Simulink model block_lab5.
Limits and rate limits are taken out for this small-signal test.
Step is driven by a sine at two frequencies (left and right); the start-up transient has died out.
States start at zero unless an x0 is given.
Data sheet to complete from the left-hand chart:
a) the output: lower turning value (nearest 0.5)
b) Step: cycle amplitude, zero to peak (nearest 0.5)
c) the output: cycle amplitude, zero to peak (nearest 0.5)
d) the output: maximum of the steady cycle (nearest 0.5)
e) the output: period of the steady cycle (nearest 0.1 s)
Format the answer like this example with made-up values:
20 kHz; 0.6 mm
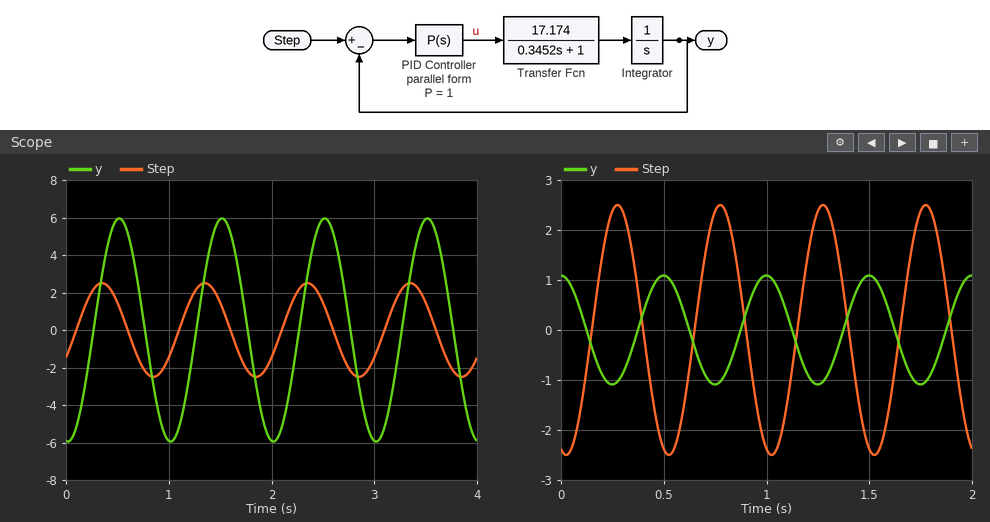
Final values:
-6.0; 2.5; 6.0; 6.0; 1.0 s
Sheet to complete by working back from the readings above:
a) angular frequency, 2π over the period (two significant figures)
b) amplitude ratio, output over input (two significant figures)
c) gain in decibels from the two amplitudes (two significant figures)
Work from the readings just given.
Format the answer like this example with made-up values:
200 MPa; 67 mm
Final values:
6.3 rad/s; 2.4; 7.6 dB
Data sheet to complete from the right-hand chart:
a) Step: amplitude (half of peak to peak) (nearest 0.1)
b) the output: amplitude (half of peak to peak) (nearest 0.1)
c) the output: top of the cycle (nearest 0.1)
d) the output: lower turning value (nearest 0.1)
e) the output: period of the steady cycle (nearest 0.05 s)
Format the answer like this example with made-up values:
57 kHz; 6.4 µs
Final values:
2.5; 1.1; 1.1; -1.1; 0.50 s
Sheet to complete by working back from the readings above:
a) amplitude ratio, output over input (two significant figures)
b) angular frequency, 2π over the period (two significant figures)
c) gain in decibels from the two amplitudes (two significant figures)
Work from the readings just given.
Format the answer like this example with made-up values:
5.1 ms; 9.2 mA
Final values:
0.44; 13 rad/s; -7.1 dB
